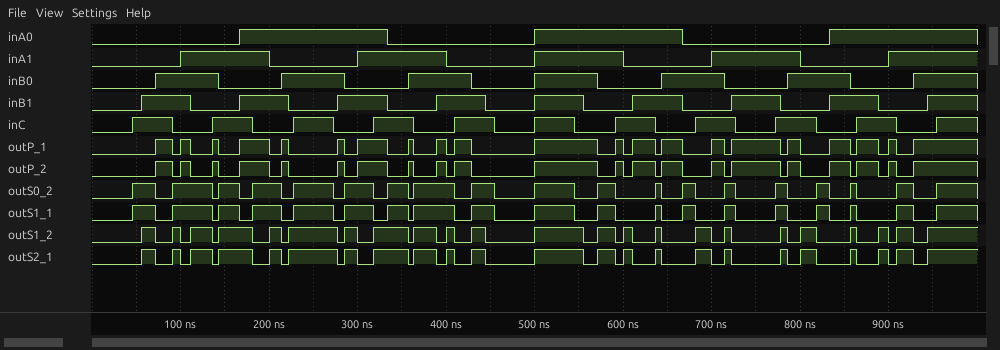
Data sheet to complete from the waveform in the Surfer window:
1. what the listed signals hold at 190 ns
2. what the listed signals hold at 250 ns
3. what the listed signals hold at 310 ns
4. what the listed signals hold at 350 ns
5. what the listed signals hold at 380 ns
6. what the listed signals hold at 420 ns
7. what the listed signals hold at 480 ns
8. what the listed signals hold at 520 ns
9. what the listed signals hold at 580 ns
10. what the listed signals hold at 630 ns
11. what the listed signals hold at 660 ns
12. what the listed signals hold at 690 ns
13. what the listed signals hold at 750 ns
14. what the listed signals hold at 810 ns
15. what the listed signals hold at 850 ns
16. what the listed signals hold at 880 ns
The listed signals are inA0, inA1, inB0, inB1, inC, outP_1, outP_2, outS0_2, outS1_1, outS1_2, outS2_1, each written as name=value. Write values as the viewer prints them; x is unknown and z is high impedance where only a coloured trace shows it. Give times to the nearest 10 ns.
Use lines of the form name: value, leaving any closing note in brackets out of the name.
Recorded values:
what the listed signals hold at 190 ns: inA0=1, inA1=1, inB0=0, inB1=1, inC=0, outP_1=1, outP_2=1, outS0_2=1, outS1_1=1, outS1_2=0, outS2_1=0
what the listed signals hold at 250 ns: inA0=1, inA1=0, inB0=1, inB1=0, inC=1, outP_1=0, outP_2=0, outS0_2=1, outS1_1=1, outS1_2=1, outS2_1=1
what the listed signals hold at 310 ns: inA0=1, inA1=1, inB0=0, inB1=1, inC=0, outP_1=1, outP_2=1, outS0_2=1, outS1_1=1, outS1_2=0, outS2_1=0
what the listed signals hold at 350 ns: inA0=0, inA1=1, inB0=0, inB1=0, inC=1, outP_1=0, outP_2=0, outS0_2=1, outS1_1=1, outS1_2=1, outS2_1=1
what the listed signals hold at 380 ns: inA0=0, inA1=1, inB0=1, inB1=0, inC=0, outP_1=0, outP_2=0, outS0_2=1, outS1_1=1, outS1_2=1, outS2_1=1
what the listed signals hold at 420 ns: inA0=0, inA1=0, inB0=1, inB1=1, inC=1, outP_1=1, outP_2=1, outS0_2=0, outS1_1=0, outS1_2=0, outS2_1=0
what the listed signals hold at 480 ns: inA0=0, inA1=0, inB0=0, inB1=0, inC=0, outP_1=0, outP_2=0, outS0_2=0, outS1_1=0, outS1_2=0, outS2_1=0
what the listed signals hold at 520 ns: inA0=1, inA1=1, inB0=1, inB1=1, inC=1, outP_1=1, outP_2=1, outS0_2=1, outS1_1=1, outS1_2=1, outS2_1=1
what the listed signals hold at 580 ns: inA0=1, inA1=1, inB0=0, inB1=0, inC=0, outP_1=0, outP_2=0, outS0_2=1, outS1_1=1, outS1_2=1, outS2_1=1
what the listed signals hold at 630 ns: inA0=1, inA1=0, inB0=0, inB1=1, inC=1, outP_1=1, outP_2=1, outS0_2=0, outS1_1=0, outS1_2=0, outS2_1=0
what the listed signals hold at 660 ns: inA0=1, inA1=0, inB0=1, inB1=1, inC=0, outP_1=1, outP_2=1, outS0_2=0, outS1_1=0, outS1_2=0, outS2_1=0
what the listed signals hold at 690 ns: inA0=0, inA1=0, inB0=1, inB1=0, inC=1, outP_1=0, outP_2=0, outS0_2=0, outS1_1=0, outS1_2=1, outS2_1=1
what the listed signals hold at 750 ns: inA0=0, inA1=1, inB0=0, inB1=1, inC=0, outP_1=1, outP_2=1, outS0_2=0, outS1_1=0, outS1_2=0, outS2_1=0
what the listed signals hold at 810 ns: inA0=0, inA1=0, inB0=1, inB1=0, inC=1, outP_1=0, outP_2=0, outS0_2=0, outS1_1=0, outS1_2=1, outS2_1=1
what the listed signals hold at 850 ns: inA0=1, inA1=0, inB0=1, inB1=1, inC=0, outP_1=1, outP_2=1, outS0_2=0, outS1_1=0, outS1_2=0, outS2_1=0
what the listed signals hold at 880 ns: inA0=1, inA1=0, inB0=0, inB1=1, inC=1, outP_1=1, outP_2=1, outS0_2=0, outS1_1=0, outS1_2=0, outS2_1=0
